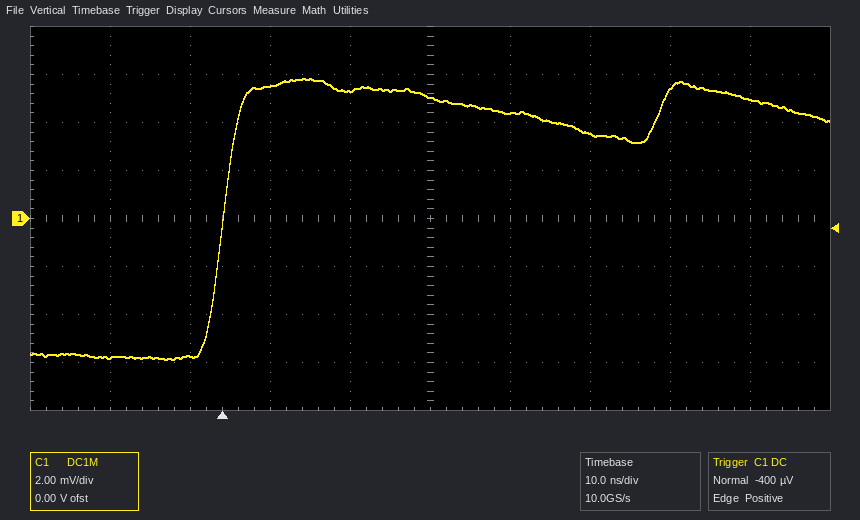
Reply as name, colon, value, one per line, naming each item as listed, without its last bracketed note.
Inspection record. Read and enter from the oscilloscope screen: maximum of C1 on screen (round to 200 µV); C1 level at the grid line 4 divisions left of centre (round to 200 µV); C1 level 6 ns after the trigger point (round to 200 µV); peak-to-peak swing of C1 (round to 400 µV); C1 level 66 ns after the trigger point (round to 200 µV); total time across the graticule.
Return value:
maximum of C1 on screen: 5.8 mV
C1 level at the grid line 4 divisions left of centre: -5.8 mV
C1 level 6 ns after the trigger point: 5.6 mV
peak-to-peak swing of C1: 11.6 mV
C1 level 66 ns after the trigger point: 5.0 mV
total time across the graticule: 100 ns
